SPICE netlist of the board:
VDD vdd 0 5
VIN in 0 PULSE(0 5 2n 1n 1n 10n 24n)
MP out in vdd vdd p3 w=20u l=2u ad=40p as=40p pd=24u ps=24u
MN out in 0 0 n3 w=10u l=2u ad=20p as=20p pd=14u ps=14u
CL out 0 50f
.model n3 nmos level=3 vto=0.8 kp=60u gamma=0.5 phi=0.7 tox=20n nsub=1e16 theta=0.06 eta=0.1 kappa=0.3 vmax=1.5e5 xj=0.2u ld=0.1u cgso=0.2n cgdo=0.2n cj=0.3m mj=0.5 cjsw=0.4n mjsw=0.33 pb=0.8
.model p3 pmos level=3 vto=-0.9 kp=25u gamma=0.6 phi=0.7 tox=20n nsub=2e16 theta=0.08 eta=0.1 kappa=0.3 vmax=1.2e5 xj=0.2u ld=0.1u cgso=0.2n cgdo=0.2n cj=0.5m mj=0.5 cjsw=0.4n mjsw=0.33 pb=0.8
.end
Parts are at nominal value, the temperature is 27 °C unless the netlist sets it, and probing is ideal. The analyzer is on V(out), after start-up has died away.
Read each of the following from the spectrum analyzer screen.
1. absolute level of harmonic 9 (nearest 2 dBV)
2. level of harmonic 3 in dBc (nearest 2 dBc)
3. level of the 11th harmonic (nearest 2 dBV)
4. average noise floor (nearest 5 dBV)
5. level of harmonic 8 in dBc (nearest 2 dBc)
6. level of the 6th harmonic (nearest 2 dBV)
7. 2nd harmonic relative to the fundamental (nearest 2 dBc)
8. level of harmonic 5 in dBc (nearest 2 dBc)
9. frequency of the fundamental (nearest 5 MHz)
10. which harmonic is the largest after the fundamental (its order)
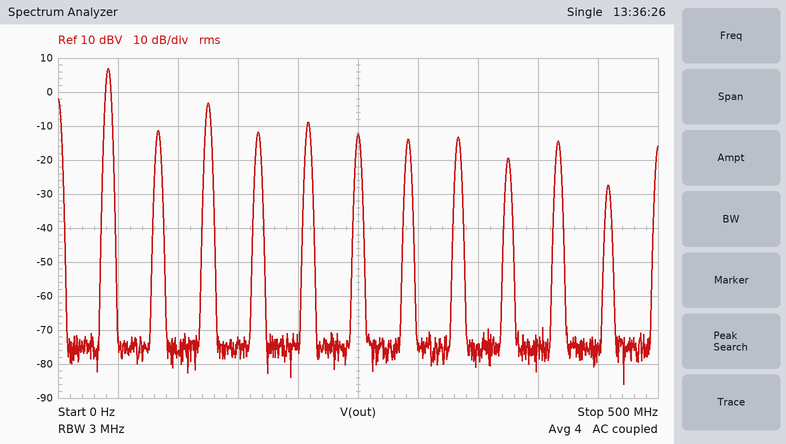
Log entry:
-20 dBV
-10 dBc
-28 dBV
-75 dBV
-20 dBc
-12 dBV
-18 dBc
-16 dBc
40 MHz
3
